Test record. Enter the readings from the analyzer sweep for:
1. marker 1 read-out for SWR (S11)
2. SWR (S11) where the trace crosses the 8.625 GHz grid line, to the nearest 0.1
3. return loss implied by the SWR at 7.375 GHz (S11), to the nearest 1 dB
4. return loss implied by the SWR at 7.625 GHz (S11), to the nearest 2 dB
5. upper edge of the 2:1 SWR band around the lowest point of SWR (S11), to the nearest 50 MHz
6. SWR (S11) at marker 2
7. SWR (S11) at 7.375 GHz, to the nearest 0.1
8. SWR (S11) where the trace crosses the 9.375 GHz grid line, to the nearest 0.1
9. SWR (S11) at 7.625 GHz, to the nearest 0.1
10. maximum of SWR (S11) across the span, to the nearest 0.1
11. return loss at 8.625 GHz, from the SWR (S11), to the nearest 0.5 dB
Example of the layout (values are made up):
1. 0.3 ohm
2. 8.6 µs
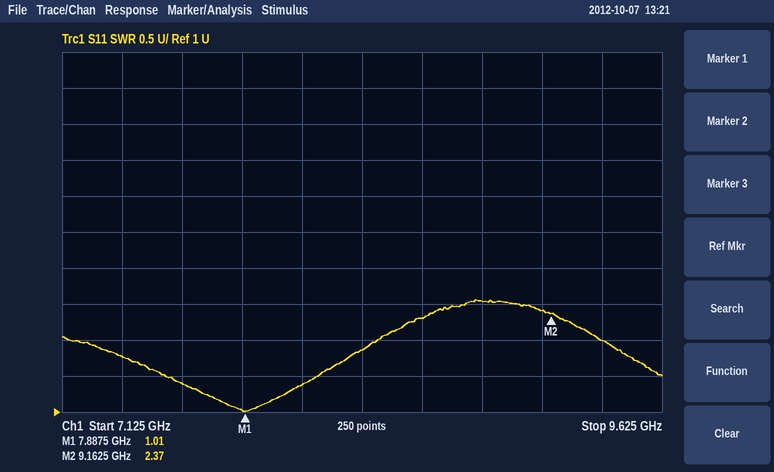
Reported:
1. 1.01
2. 2.3
3. 11 dB
4. 16 dB
5. 8.45 GHz
6. 2.37
7. 1.8
8. 2.0
9. 1.4
10. 2.6
11. 8.0 dB
